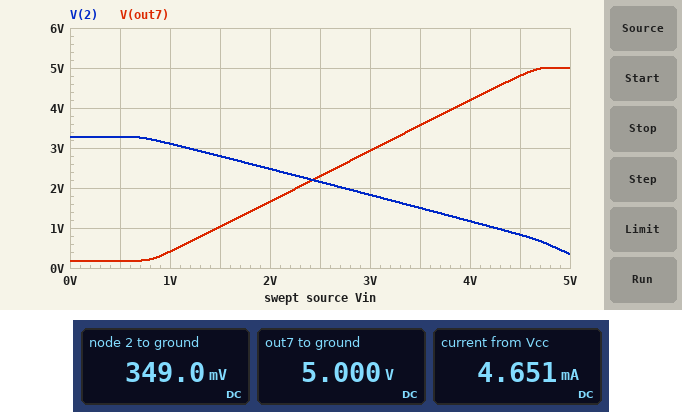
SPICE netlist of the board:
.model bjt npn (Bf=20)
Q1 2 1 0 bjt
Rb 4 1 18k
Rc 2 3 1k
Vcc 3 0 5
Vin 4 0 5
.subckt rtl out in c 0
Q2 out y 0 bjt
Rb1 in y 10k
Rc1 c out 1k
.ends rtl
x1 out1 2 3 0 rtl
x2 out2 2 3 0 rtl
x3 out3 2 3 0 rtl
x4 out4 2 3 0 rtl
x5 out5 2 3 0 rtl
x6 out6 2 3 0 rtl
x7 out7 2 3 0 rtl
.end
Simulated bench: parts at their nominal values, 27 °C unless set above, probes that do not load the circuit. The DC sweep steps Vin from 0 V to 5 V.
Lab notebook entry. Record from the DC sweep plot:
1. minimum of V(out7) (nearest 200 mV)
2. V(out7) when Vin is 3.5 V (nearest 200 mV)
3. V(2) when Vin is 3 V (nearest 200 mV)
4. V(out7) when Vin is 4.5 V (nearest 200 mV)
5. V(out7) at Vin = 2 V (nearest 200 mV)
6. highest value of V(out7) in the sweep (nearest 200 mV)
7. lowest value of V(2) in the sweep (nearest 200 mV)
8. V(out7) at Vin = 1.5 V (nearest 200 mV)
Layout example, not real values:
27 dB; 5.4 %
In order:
200 mV; 3.6 V; 1.8 V; 4.8 V; 1.6 V; 5.0 V; 400 mV; 1.0 V
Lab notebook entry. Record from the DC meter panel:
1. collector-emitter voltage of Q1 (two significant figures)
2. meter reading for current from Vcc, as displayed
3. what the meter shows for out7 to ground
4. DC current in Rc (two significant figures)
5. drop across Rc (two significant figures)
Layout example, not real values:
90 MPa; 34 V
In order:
350 mV; 4.651 mA; 5.000 V; 4.7 mA; 4.7 V
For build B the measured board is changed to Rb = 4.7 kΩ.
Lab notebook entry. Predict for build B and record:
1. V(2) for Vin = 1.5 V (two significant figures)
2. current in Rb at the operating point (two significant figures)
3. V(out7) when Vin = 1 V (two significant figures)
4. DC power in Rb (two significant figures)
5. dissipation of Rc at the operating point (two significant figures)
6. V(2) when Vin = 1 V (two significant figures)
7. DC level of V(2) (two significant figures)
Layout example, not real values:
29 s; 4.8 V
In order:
1.5 V; 890 µA; 1.2 V; 3.7 mW; 24 mW; 2.7 V; 61 mV
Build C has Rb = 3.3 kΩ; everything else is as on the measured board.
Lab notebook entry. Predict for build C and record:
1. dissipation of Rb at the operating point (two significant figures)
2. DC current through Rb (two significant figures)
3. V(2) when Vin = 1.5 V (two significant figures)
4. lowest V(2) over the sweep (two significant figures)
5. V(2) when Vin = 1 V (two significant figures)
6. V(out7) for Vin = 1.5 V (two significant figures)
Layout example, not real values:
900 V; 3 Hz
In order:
5.3 mW; 1.3 mA; 780 mV; 52 mV; 2.5 V; 4.9 V
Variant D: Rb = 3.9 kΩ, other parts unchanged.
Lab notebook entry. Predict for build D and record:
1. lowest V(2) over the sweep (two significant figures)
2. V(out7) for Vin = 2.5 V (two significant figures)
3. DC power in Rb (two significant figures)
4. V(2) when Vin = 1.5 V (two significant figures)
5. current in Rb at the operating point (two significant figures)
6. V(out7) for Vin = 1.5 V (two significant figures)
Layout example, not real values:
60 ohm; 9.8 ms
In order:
56 mV; 5.0 V; 4.5 mW; 1.2 V; 1.1 mA; 4.2 V
